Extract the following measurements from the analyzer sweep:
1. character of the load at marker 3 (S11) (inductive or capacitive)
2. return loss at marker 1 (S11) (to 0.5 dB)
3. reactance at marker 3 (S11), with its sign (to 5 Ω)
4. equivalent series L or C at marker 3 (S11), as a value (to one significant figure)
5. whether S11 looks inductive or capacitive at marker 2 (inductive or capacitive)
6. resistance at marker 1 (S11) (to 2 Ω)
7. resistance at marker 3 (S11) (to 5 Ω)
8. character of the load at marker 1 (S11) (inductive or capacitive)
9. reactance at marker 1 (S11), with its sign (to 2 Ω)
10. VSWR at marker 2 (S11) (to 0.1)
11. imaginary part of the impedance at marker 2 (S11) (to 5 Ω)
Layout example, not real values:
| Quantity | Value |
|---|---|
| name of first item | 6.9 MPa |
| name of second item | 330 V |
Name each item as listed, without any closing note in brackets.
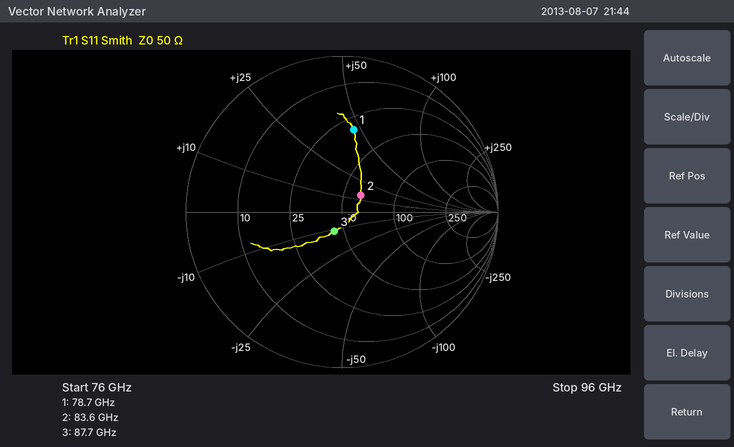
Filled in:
| Quantity | Value |
|---|---|
| character of the load at marker 3 (S11) | capacitive |
| return loss at marker 1 (S11) | 5.5 dB |
| reactance at marker 3 (S11), with its sign | -10 Ω |
| equivalent series L or C at marker 3 (S11), as a value | 200 fF |
| whether S11 looks inductive or capacitive at marker 2 | inductive |
| resistance at marker 1 (S11) | 32 Ω |
| resistance at marker 3 (S11) | 45 Ω |
| character of the load at marker 1 (S11) | inductive |
| reactance at marker 1 (S11), with its sign | +46 Ω |
| VSWR at marker 2 (S11) | 1.4 |
| imaginary part of the impedance at marker 2 (S11) | +15 Ω |
